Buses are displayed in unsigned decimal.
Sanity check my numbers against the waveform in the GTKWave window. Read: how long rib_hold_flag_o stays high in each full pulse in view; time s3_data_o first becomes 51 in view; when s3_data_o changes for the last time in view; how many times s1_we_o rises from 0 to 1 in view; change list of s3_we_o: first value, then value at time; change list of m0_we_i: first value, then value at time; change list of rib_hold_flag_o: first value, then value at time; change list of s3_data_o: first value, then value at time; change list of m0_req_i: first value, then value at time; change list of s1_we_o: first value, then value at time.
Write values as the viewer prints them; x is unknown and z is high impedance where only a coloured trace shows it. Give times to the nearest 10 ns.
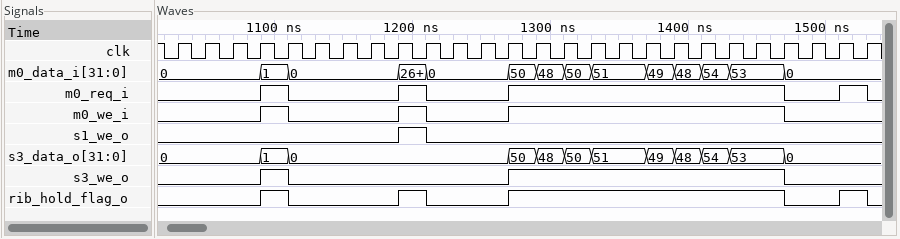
20 ns, 20 ns, 200 ns, 20 ns
1330 ns
1470 ns
1
0, 1 at 1090 ns, 0 at 1110 ns, 1 at 1270 ns, 0 at 1470 ns
0, 1 at 1090 ns, 0 at 1110 ns, 1 at 1190 ns, 0 at 1210 ns, 1 at 1270 ns, 0 at 1470 ns
0, 1 at 1090 ns, 0 at 1110 ns, 1 at 1190 ns, 0 at 1210 ns, 1 at 1270 ns, 0 at 1470 ns, 1 at 1510 ns, 0 at 1530 ns
0, 1 at 1090 ns, 0 at 1110 ns, 50 at 1270 ns, 48 at 1290 ns, 50 at 1310 ns, 51 at 1330 ns, 49 at 1370 ns, 48 at 1390 ns, 54 at 1410 ns, 53 at 1430 ns, 0 at 1470 ns
0, 1 at 1090 ns, 0 at 1110 ns, 1 at 1190 ns, 0 at 1210 ns, 1 at 1270 ns, 0 at 1470 ns, 1 at 1510 ns, 0 at 1530 ns
0, 1 at 1190 ns, 0 at 1210 ns
